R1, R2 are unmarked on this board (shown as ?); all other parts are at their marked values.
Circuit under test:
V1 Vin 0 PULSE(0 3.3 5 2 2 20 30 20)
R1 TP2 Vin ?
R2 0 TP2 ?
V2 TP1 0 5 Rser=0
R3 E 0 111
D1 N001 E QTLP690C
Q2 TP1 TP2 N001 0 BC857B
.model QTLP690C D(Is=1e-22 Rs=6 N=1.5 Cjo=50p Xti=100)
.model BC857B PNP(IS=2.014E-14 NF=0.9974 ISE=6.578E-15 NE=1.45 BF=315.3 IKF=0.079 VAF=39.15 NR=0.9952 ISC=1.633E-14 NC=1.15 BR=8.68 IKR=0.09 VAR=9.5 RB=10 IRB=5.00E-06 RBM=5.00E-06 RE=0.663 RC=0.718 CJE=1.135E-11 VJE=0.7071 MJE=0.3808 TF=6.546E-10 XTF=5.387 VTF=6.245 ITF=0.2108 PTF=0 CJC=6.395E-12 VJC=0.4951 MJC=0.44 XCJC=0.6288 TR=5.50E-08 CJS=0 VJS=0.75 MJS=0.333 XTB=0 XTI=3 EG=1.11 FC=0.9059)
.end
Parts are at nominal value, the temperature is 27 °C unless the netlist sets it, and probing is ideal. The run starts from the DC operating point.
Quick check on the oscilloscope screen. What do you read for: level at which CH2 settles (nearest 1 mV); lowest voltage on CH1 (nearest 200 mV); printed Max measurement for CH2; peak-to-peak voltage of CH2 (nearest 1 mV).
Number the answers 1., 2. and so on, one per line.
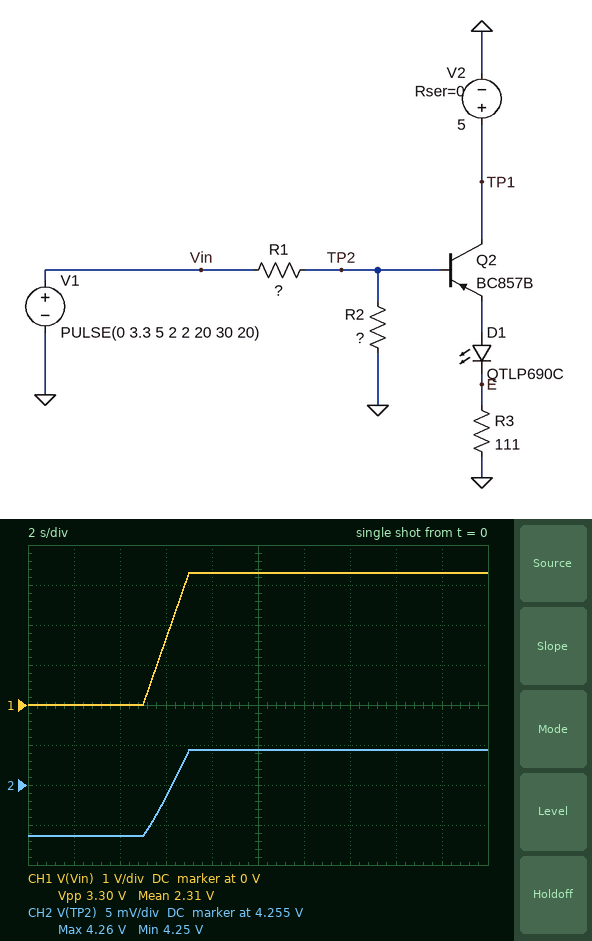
1. 4.259 V
2. 0 V
3. 4.26 V
4. 11 mV
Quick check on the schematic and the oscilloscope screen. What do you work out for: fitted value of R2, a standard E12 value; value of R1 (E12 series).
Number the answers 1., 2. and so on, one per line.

1. 1.2 kΩ
2. 2.7 kΩ
